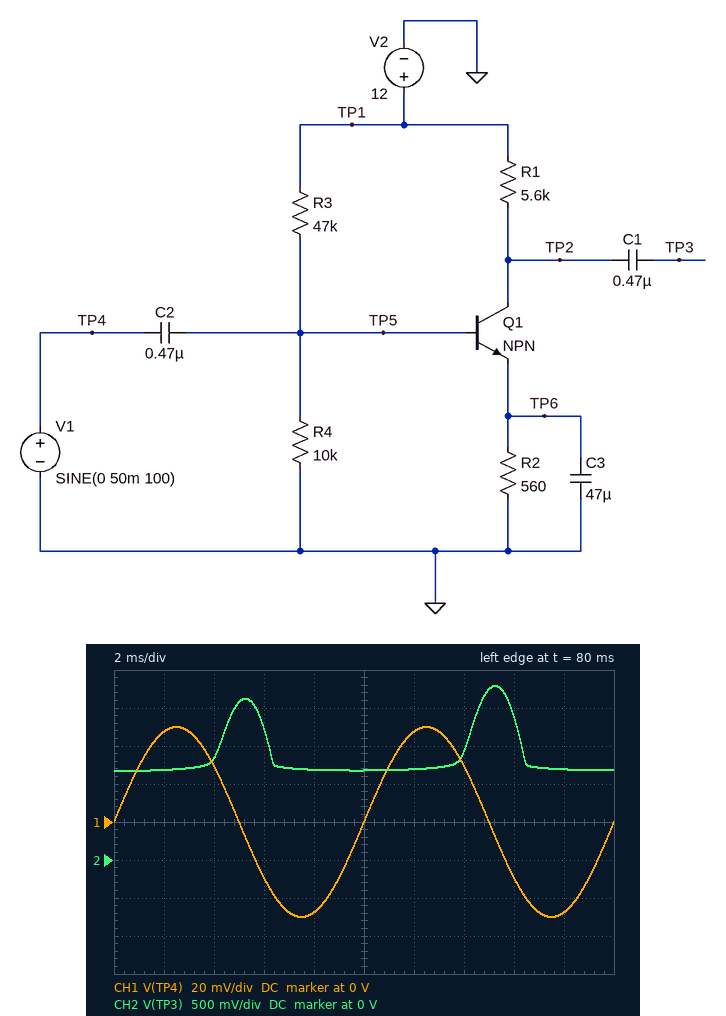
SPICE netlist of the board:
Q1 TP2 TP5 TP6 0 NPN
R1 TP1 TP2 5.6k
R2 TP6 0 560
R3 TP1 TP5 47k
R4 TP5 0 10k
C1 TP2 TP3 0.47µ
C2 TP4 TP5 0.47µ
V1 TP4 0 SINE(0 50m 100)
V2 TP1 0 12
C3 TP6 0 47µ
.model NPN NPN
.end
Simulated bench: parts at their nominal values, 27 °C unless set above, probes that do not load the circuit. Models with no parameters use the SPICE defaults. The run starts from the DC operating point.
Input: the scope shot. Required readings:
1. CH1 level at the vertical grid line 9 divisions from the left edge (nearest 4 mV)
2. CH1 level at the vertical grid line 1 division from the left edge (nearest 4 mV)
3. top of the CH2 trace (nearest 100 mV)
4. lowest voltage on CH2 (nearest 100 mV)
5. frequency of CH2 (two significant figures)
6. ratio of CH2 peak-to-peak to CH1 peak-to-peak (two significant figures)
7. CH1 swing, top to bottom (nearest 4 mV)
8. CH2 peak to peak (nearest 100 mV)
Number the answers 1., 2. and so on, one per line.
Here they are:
1. -48 mV
2. 48 mV
3. 2.3 V
4. 1.2 V
5. 100 Hz
6. 11
7. 100 mV
8. 1.1 V
